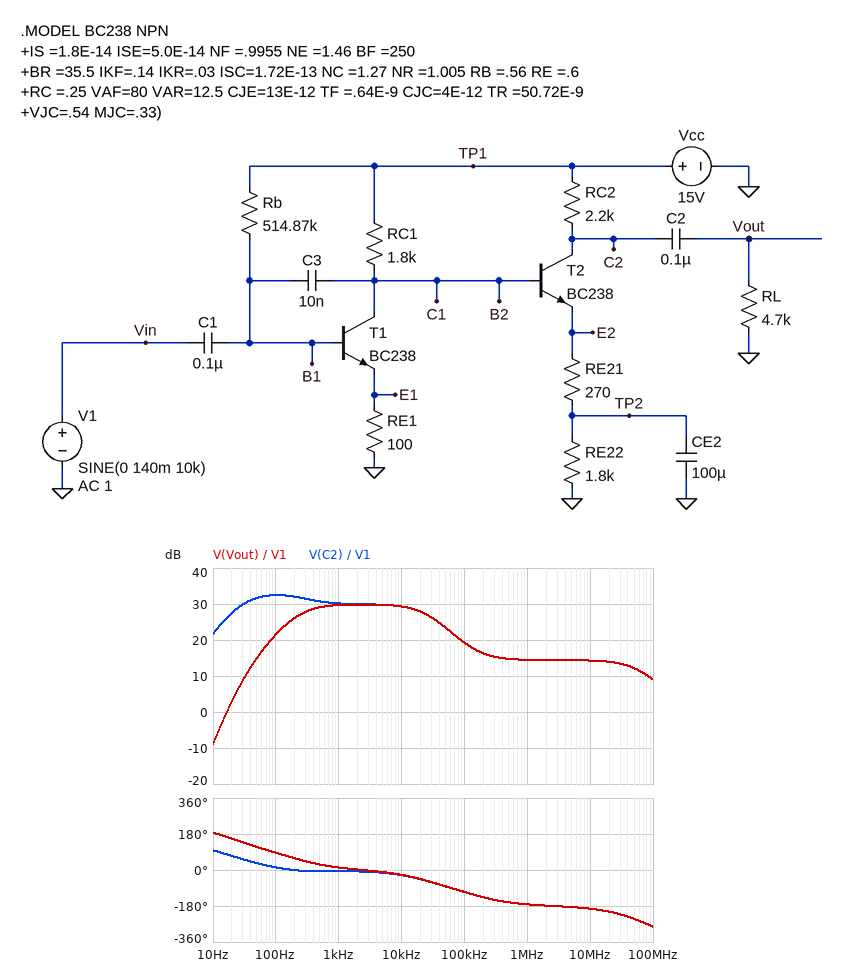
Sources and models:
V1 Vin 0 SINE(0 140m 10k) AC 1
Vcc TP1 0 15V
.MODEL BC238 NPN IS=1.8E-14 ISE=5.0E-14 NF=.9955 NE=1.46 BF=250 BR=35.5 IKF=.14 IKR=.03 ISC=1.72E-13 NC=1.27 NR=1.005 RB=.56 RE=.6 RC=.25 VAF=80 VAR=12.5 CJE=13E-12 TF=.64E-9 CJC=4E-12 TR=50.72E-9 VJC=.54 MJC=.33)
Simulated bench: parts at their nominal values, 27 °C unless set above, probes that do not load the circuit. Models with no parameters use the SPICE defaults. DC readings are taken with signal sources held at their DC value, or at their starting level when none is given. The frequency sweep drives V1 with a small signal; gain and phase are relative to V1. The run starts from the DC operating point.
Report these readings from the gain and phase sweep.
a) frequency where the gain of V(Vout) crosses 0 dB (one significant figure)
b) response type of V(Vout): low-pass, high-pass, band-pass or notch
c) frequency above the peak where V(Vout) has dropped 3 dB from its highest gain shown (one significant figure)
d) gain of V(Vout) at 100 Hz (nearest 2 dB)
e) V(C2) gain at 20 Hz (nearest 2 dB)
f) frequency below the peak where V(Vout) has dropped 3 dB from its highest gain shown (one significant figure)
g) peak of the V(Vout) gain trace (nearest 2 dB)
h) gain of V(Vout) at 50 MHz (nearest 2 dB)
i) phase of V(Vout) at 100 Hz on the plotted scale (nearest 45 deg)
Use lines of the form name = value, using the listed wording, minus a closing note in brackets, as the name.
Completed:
frequency where the gain of V(Vout) crosses 0 dB = 20 Hz
response type of V(Vout): low-pass, high-pass, band-pass or notch = band-pass
frequency above the peak where V(Vout) has dropped 3 dB from its highest gain shown = 30 kHz
gain of V(Vout) at 100 Hz = 22 dB
V(C2) gain at 20 Hz = 28 dB
frequency below the peak where V(Vout) has dropped 3 dB from its highest gain shown = 200 Hz
peak of the V(Vout) gain trace = 30 dB
gain of V(Vout) at 50 MHz = 12 dB
phase of V(Vout) at 100 Hz on the plotted scale = 90 deg
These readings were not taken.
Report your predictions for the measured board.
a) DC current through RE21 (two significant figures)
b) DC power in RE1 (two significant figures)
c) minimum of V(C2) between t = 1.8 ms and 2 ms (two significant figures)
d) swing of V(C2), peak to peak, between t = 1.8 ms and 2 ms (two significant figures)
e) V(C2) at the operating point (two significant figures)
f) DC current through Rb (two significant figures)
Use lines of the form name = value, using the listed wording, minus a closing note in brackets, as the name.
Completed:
DC current through RE21 = 2.1 mA
DC power in RE1 = 3.1 mW
minimum of V(C2) between t = 1.8 ms and 2 ms = 6.2 V
swing of V(C2), peak to peak, between t = 1.8 ms and 2 ms = 7.3 V
V(C2) at the operating point = 10 V
DC current through Rb = 27 µA
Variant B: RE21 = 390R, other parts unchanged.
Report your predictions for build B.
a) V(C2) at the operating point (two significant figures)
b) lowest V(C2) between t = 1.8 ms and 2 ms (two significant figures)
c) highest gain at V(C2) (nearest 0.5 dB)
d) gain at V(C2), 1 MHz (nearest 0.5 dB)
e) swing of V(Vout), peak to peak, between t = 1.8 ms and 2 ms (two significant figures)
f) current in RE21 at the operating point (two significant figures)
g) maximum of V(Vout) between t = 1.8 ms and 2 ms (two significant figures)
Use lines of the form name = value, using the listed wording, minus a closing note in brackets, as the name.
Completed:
V(C2) at the operating point = 11 V
lowest V(C2) between t = 1.8 ms and 2 ms = 7.7 V
highest gain at V(C2) = 29.5 dB
gain at V(C2), 1 MHz = 11.5 dB
swing of V(Vout), peak to peak, between t = 1.8 ms and 2 ms = 5.6 V
current in RE21 at the operating point = 2.0 mA
maximum of V(Vout) between t = 1.8 ms and 2 ms = 2.8 V
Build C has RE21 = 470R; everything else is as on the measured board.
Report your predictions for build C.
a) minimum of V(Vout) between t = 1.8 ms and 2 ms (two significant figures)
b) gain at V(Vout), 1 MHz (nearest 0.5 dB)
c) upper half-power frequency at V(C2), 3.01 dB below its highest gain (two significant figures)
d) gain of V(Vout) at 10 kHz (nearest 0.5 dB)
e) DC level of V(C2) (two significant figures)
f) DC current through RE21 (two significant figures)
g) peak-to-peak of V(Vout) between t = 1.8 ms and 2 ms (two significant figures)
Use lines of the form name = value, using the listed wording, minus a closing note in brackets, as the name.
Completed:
minimum of V(Vout) between t = 1.8 ms and 2 ms = -2.4 V
gain at V(Vout), 1 MHz = 10.0 dB
upper half-power frequency at V(C2), 3.01 dB below its highest gain = 8.5 kHz
gain of V(Vout) at 10 kHz = 24.5 dB
DC level of V(C2) = 11 V
DC current through RE21 = 1.9 mA
peak-to-peak of V(Vout) between t = 1.8 ms and 2 ms = 4.8 V
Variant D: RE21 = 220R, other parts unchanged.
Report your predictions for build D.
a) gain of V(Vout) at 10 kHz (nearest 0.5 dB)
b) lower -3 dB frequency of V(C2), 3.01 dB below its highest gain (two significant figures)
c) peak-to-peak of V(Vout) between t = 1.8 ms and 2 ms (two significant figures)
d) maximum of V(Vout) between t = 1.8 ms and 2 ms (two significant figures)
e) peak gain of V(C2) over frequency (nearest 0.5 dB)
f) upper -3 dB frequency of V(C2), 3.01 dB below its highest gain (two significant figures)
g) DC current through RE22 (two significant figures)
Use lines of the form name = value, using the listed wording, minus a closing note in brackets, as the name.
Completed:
gain of V(Vout) at 10 kHz = 31.0 dB
lower -3 dB frequency of V(C2), 3.01 dB below its highest gain = 28 Hz
peak-to-peak of V(Vout) between t = 1.8 ms and 2 ms = 8.2 V
maximum of V(Vout) between t = 1.8 ms and 2 ms = 3.6 V
peak gain of V(C2) over frequency = 34.0 dB
upper -3 dB frequency of V(C2), 3.01 dB below its highest gain = 8.8 kHz
DC current through RE22 = 2.2 mA
